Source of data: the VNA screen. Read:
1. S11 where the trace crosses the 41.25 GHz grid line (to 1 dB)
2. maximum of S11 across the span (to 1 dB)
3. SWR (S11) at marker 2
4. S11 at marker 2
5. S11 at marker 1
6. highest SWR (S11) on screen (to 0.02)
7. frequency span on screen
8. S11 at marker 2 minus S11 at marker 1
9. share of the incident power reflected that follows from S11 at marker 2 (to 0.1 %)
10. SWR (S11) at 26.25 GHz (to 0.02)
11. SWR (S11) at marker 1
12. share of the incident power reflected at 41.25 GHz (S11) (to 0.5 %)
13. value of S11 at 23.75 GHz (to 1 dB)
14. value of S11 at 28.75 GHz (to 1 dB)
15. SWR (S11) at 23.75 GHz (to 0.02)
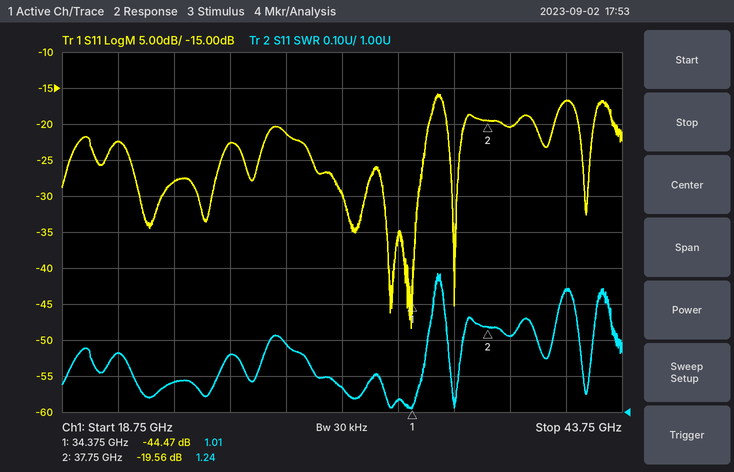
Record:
-17 dB
-16 dB
1.24
-19.56 dB
-44.47 dB
1.38
25 GHz
24.91 dB
1.1 %
1.16
1.01
2.0 %
-28 dB
-21 dB
1.08
